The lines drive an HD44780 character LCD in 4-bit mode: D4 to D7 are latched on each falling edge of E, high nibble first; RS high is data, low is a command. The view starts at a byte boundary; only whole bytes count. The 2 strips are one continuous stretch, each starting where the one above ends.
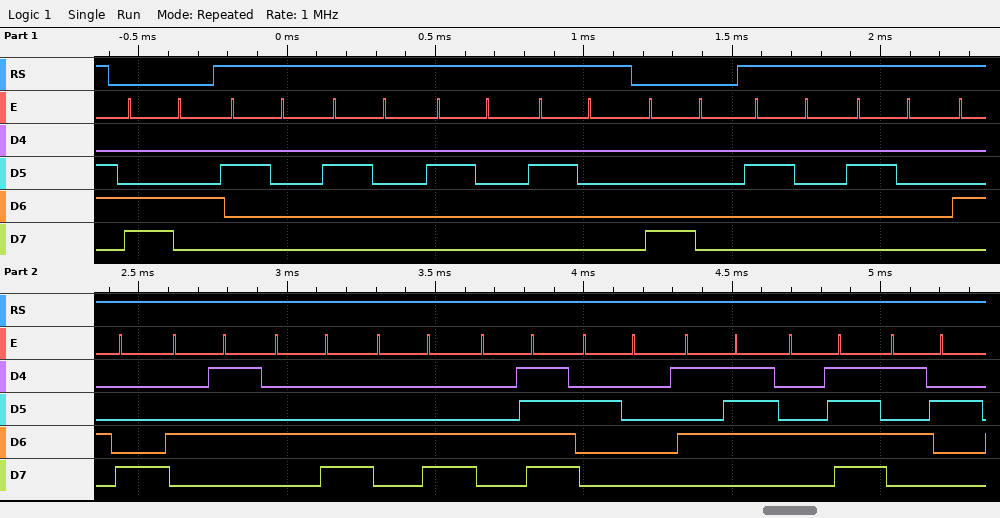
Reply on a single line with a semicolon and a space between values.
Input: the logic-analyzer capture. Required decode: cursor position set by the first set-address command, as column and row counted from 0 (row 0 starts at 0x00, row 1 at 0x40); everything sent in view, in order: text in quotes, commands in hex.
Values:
column 4, row 1; 0xC4 "    " 0x80 "  HELLO WOR"
